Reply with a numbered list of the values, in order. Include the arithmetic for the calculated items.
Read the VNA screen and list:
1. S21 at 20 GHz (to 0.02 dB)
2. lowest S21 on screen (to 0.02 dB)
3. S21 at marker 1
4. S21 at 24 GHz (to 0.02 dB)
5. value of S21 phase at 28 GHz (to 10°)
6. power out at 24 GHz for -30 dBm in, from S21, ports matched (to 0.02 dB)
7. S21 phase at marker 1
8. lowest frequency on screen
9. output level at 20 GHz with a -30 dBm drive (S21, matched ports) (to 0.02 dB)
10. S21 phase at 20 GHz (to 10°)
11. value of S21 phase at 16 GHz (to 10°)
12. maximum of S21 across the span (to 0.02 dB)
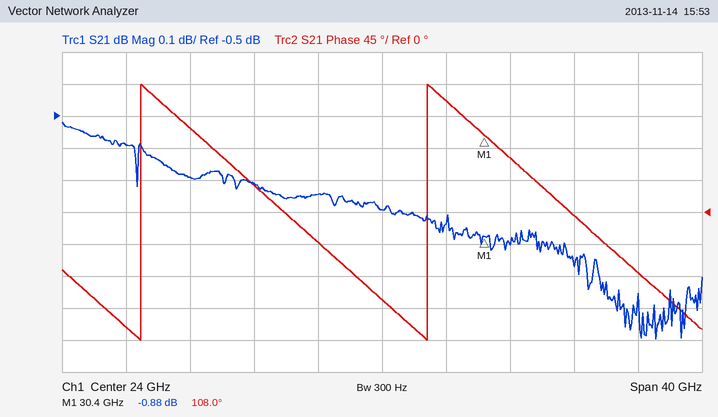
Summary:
1. -0.74 dB
2. -1.20 dB
3. -0.88 dB
4. -0.80 dB
5. 160°
6. -30 dBm + (-0.80 dB) = -30.80 dBm
7. 108.0°
8. 4 GHz
9. -30 dBm + (-0.74 dB) = -30.74 dBm
10. -40°
11. 40°
12. -0.52 dB
